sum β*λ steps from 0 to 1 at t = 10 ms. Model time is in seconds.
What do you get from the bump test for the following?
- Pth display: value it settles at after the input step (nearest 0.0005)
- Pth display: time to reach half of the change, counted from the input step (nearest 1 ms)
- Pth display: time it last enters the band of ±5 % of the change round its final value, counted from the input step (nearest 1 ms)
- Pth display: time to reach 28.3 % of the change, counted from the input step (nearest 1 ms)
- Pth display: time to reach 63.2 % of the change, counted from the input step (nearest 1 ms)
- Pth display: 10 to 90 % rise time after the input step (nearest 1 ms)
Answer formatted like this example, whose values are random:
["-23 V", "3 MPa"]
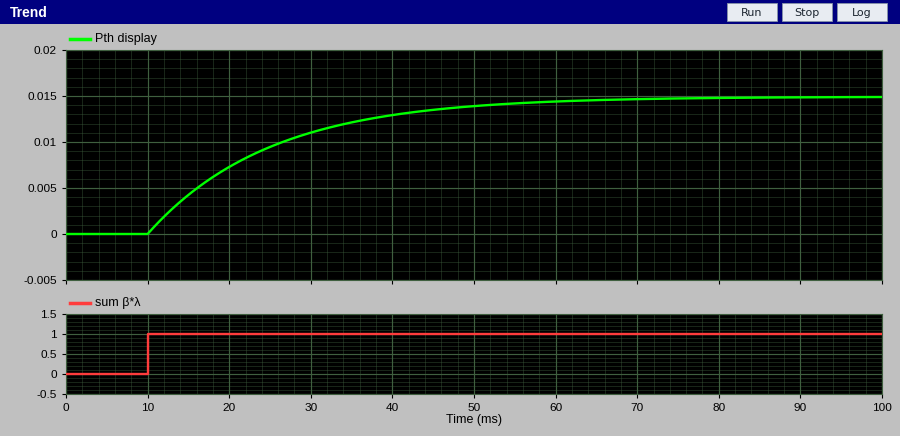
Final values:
["0.0150", "10 ms", "45 ms", "5 ms", "15 ms", "33 ms"]
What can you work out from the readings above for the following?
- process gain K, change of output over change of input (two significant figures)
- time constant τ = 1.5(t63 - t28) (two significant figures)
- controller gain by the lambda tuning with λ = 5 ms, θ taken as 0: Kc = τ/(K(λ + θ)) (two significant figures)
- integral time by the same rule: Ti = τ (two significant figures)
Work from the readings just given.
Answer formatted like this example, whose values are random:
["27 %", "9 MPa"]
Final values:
["0.015", "15 ms", "200", "15 ms"]
